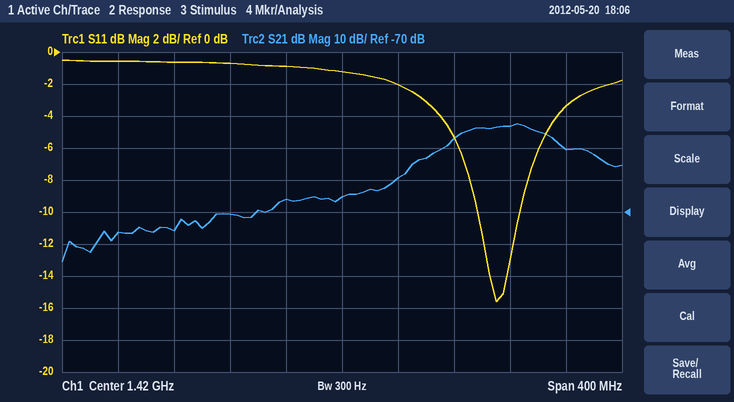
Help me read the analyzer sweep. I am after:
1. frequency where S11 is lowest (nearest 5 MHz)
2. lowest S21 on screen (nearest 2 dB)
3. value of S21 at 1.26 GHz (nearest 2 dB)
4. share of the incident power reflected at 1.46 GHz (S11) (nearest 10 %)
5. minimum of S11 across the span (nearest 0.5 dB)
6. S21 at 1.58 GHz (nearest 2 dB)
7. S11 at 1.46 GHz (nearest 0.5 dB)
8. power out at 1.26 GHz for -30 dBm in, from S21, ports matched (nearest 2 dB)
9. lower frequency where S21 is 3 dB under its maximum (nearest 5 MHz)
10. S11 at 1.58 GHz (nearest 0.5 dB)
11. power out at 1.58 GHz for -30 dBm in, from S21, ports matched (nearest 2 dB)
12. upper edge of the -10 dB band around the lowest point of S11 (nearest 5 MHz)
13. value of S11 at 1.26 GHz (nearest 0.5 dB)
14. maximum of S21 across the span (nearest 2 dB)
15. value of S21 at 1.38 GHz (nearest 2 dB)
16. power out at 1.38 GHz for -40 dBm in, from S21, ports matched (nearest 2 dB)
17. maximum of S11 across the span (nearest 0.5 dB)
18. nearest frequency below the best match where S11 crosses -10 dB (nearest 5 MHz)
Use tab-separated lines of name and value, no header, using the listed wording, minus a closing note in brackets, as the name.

frequency where S11 is lowest	1.530 GHz
lowest S21 on screen	-86 dB
value of S21 at 1.26 GHz	-76 dB
share of the incident power reflected at 1.46 GHz (S11)	60 %
minimum of S11 across the span	-15.5 dB
S21 at 1.58 GHz	-50 dB
S11 at 1.46 GHz	-2.0 dB
power out at 1.26 GHz for -30 dBm in, from S21, ports matched	-106 dBm
lower frequency where S21 is 3 dB under its maximum	1.505 GHz
S11 at 1.58 GHz	-3.5 dB
power out at 1.58 GHz for -30 dBm in, from S21, ports matched	-80 dBm
upper edge of the -10 dB band around the lowest point of S11	1.545 GHz
value of S11 at 1.26 GHz	-0.5 dB
maximum of S21 across the span	-42 dB
value of S21 at 1.38 GHz	-66 dB
power out at 1.38 GHz for -40 dBm in, from S21, ports matched	-106 dBm
maximum of S11 across the span	-0.5 dB
nearest frequency below the best match where S11 crosses -10 dB	1.515 GHz
